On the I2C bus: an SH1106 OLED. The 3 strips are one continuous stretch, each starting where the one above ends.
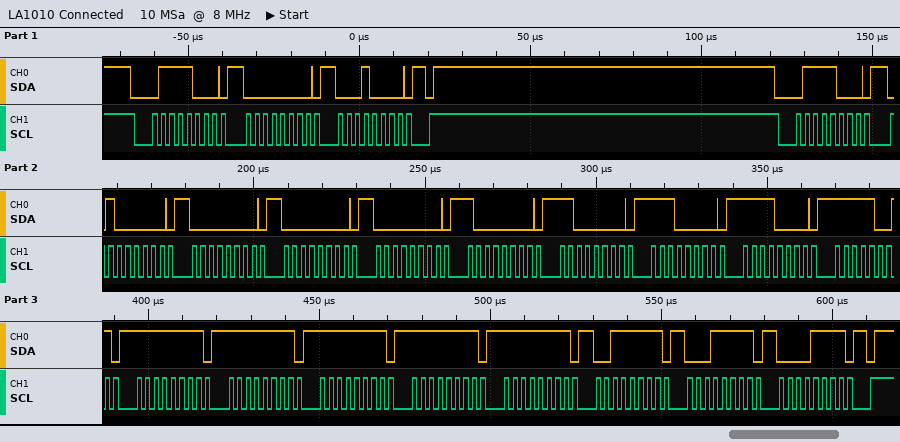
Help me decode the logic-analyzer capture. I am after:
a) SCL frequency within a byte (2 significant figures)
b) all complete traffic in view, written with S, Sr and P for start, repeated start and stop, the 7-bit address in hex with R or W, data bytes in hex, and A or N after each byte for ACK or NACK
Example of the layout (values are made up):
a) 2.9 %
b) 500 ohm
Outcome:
a) 400 kHz
b) S 3CW A 00 A 10 A P S 3CW A 40 A 00 A 00 A 00 A 80 A C0 A E0 A F0 A F9 A FF A FF A FF A FF A FF A 3F A 1F A 0F A P
